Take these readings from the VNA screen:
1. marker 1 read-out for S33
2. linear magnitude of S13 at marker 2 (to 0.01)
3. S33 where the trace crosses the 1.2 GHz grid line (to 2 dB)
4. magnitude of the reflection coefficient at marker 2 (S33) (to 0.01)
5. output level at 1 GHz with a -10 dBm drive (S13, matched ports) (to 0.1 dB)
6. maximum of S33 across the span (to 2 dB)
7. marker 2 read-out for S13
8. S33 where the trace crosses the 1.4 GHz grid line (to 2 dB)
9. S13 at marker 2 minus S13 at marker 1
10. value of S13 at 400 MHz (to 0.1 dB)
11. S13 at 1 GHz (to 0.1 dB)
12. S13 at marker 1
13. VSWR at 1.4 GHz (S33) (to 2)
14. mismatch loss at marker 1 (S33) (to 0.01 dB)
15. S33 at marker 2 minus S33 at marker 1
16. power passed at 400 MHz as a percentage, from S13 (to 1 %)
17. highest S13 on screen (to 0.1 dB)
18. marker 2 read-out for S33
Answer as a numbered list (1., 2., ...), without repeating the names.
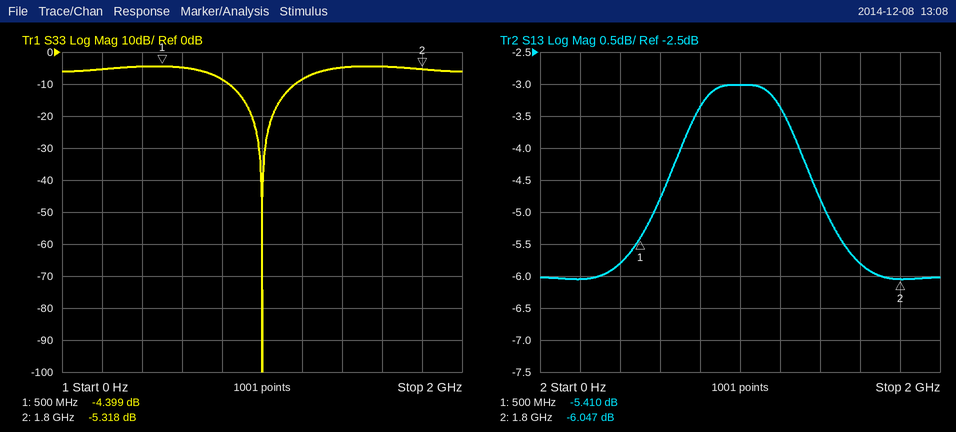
1. -4.399 dB
2. 0.50
3. -8 dB
4. 0.54
5. -13.0 dBm
6. -4 dB
7. -6.047 dB
8. -4 dB
9. -0.637 dB
10. -5.8 dB
11. -3.0 dB
12. -5.410 dB
13. 4
14. 1.96 dB
15. -0.919 dB
16. 26 %
17. -3.0 dB
18. -5.318 dB
